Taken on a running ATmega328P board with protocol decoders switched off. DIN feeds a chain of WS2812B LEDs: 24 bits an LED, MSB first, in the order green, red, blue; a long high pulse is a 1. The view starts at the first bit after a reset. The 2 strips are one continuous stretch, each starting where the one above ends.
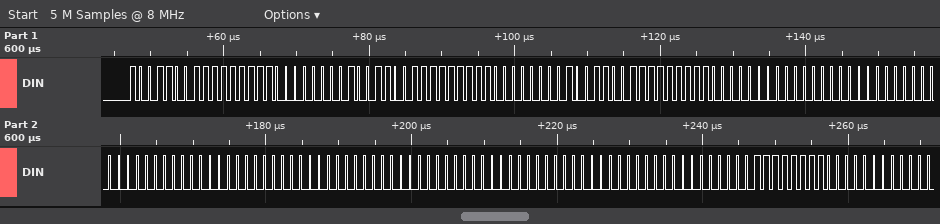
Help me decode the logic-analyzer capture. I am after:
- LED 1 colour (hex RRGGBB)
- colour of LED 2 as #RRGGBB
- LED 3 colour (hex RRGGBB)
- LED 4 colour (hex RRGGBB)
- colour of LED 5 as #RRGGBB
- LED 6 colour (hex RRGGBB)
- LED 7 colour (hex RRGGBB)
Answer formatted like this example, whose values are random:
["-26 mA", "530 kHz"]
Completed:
["#FF9900", "#FF9900", "#FF9900", "#000000", "#000000", "#000000", "#0000FF"]
